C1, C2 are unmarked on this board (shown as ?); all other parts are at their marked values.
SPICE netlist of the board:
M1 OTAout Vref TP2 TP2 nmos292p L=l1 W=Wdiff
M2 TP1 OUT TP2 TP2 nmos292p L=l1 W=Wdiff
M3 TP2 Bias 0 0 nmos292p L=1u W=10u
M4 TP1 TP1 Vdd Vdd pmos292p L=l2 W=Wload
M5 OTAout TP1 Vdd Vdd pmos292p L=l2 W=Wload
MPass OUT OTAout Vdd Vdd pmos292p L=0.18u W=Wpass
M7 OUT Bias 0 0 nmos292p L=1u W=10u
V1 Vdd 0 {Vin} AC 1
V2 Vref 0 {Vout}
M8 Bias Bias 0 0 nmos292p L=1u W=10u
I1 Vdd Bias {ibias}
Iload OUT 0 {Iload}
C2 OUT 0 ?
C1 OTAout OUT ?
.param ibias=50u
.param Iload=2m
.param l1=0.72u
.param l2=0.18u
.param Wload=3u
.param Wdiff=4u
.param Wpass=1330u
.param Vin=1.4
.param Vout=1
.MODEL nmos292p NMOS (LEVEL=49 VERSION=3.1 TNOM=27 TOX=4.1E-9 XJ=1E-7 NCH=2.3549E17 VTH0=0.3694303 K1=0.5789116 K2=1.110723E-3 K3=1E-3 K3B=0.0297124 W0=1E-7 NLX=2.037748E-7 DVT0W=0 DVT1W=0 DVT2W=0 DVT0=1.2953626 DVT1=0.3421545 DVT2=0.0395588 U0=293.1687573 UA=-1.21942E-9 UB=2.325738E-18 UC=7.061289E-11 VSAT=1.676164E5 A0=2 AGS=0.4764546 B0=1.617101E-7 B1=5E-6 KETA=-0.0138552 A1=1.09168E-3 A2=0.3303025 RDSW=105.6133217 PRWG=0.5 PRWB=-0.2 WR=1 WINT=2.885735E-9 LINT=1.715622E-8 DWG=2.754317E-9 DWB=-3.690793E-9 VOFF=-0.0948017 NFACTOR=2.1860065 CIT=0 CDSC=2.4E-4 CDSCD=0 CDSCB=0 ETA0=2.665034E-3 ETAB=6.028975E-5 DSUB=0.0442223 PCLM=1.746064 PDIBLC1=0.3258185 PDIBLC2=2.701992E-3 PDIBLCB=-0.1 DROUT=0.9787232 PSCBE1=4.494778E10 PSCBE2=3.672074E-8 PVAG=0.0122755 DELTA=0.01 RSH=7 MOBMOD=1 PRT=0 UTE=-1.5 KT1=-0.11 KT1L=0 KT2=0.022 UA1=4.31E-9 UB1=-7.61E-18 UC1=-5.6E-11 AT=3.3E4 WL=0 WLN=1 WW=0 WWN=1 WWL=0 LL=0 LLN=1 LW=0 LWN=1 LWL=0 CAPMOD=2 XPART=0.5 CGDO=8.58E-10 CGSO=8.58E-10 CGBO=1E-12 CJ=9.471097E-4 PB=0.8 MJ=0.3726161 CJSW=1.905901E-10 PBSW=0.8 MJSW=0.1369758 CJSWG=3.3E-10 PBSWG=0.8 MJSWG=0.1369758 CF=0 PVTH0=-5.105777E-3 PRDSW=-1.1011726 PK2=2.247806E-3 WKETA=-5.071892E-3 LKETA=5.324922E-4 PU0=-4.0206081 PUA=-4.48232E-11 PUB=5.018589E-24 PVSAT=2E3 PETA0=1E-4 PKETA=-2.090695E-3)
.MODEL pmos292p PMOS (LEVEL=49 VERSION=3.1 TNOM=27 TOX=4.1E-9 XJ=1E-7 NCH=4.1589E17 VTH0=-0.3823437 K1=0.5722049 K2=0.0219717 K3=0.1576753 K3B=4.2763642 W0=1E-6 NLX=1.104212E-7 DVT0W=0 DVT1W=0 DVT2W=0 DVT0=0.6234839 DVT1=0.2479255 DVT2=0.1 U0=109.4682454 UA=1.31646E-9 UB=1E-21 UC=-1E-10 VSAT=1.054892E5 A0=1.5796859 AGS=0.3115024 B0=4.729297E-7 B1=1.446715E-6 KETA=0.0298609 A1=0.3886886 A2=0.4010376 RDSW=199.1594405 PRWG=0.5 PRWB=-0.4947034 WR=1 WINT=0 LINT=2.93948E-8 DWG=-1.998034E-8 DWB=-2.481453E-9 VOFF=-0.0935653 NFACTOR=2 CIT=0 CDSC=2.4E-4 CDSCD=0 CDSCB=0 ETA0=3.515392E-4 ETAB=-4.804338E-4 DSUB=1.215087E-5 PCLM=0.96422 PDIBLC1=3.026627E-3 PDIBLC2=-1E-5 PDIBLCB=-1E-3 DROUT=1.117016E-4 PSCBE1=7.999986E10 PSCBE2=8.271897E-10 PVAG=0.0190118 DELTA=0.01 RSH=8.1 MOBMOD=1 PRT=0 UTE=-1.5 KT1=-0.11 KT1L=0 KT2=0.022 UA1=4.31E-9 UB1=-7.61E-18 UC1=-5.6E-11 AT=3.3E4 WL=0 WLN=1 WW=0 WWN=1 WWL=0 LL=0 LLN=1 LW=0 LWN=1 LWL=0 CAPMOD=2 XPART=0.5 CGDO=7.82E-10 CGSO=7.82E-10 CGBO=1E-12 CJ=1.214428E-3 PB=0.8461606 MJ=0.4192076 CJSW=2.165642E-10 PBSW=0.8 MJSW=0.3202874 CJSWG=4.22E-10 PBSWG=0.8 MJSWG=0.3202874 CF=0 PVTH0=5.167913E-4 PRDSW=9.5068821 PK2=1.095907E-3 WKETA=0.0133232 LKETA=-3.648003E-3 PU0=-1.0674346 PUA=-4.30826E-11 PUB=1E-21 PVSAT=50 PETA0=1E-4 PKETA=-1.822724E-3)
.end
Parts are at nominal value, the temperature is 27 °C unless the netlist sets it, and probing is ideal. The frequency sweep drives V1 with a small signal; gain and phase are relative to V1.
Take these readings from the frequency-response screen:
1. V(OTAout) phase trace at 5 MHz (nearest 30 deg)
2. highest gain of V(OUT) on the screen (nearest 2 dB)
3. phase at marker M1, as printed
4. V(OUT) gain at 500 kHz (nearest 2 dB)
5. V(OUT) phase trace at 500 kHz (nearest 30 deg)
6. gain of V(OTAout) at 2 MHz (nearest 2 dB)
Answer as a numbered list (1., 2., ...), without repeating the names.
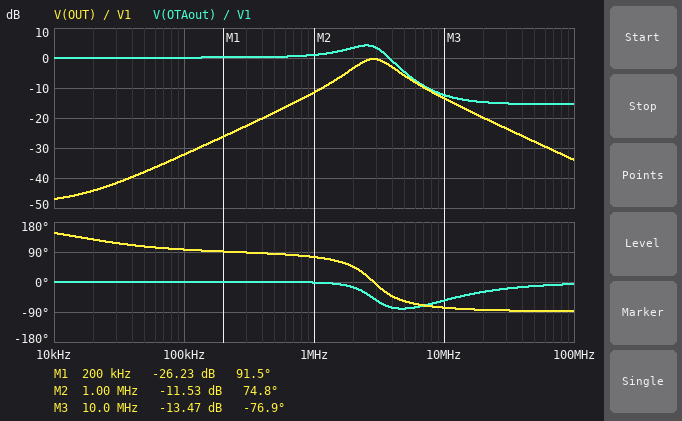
1. -90 deg
2. 0 dB
3. 91.5 deg
4. -18 dB
5. 90 deg
6. 4 dB
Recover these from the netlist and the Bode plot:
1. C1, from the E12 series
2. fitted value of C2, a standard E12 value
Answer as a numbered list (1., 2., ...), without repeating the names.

1. 8.2 pF
2. 1.8 nF
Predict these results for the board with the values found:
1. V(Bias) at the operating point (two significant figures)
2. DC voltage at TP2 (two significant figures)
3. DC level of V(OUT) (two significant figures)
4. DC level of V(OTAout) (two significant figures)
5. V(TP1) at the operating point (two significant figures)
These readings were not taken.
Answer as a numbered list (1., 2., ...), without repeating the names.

1. 620 mV
2. 380 mV
3. 1.0 V
4. 840 mV
5. 750 mV
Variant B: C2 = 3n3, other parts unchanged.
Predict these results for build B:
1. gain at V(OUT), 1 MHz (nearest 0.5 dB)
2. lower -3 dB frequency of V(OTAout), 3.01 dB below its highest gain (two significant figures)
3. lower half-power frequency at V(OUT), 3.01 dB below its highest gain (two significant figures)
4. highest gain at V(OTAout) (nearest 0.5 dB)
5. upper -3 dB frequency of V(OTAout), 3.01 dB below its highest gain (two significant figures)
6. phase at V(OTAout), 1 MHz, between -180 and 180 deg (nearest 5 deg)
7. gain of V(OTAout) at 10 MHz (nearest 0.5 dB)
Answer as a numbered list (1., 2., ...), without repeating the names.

1. -10.5 dB
2. 1.2 MHz
3. 1.6 MHz
4. 5.5 dB
5. 2.5 MHz
6. -5 deg
7. -15.0 dB
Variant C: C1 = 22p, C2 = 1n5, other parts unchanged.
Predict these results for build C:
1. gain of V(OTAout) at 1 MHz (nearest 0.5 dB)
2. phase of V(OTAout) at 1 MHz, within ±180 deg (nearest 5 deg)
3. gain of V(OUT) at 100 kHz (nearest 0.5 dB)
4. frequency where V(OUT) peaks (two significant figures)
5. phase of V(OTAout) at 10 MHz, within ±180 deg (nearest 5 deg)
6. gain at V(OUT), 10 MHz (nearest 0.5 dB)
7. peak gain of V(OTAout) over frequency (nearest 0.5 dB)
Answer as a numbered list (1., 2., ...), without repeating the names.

1. 1.5 dB
2. -5 deg
3. -24.5 dB
4. 2.1 MHz
5. -70 deg
6. -11.5 dB
7. 2.5 dB
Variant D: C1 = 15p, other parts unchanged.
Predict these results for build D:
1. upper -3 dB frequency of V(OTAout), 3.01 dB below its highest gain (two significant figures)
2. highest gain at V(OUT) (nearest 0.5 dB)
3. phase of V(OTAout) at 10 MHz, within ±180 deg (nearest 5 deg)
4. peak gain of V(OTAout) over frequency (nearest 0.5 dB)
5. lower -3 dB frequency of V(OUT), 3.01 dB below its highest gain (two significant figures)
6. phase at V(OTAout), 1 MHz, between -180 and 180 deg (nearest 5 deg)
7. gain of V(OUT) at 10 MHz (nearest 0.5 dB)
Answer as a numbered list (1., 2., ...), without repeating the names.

1. 3.0 MHz
2. 0 dB
3. -65 deg
4. 3.0 dB
5. 1.4 MHz
6. -5 deg
7. -13.0 dB
